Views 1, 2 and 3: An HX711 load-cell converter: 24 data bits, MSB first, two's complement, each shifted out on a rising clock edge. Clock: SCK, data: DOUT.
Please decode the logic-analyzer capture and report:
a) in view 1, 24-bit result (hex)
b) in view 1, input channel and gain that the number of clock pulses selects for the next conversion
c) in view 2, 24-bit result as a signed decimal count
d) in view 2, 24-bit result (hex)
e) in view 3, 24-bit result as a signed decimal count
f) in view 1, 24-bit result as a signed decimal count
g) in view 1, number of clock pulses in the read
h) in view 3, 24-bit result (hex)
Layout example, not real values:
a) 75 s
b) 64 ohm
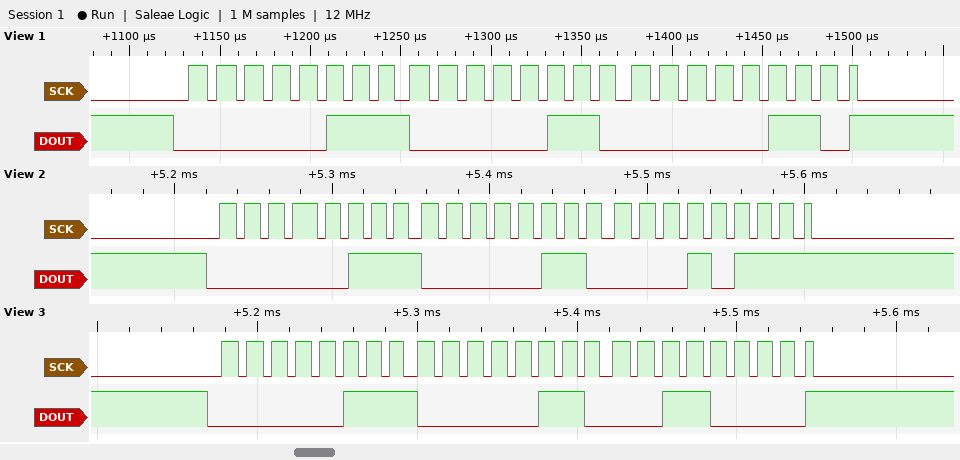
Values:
a) 0x070606
b) channel A, gain 128
c) 460311
d) 0x070617
e) 460336
f) 460294
g) 25
h) 0x070630
